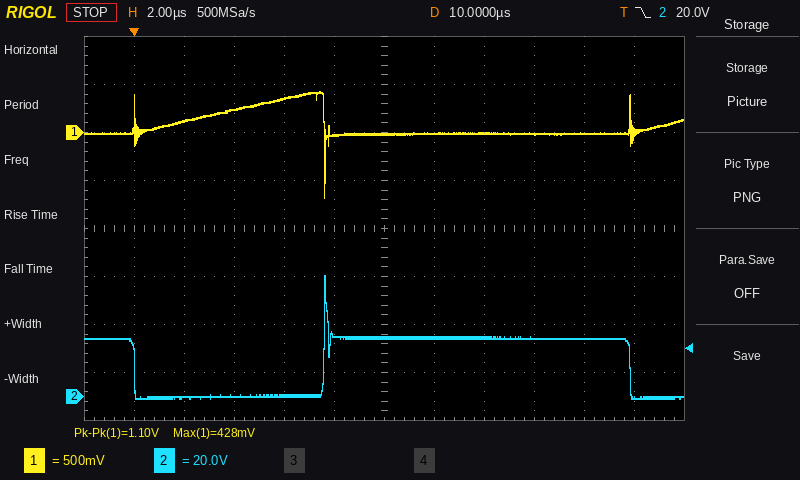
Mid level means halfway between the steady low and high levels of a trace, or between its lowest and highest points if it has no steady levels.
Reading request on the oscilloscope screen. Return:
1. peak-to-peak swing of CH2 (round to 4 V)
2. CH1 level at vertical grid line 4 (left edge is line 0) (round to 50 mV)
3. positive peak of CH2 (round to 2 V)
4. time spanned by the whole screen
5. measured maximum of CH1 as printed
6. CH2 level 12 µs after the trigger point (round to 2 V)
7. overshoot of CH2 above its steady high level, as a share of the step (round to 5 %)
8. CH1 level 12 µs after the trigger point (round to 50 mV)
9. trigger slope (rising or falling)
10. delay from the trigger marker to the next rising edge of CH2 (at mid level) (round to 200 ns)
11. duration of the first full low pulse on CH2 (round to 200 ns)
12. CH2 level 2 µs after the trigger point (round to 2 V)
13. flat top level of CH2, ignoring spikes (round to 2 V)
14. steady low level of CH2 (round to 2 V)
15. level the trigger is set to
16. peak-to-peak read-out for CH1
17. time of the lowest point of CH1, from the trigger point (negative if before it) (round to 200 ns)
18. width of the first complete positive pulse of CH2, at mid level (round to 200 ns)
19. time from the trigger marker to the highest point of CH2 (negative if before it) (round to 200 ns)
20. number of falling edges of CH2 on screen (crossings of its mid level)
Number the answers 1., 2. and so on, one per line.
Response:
1. 52 V
2. 350 mV
3. 50 V
4. 24 µs
5. 428 mV
6. 24 V
7. 105 %
8. 0 mV
9. falling
10. 7.6 µs
11. 7.6 µs
12. 0 V
13. 24 V
14. 0 V
15. 20.0 V
16. 1.10 V
17. +7.6 µs
18. 12.2 µs
19. +7.6 µs
20. 2
